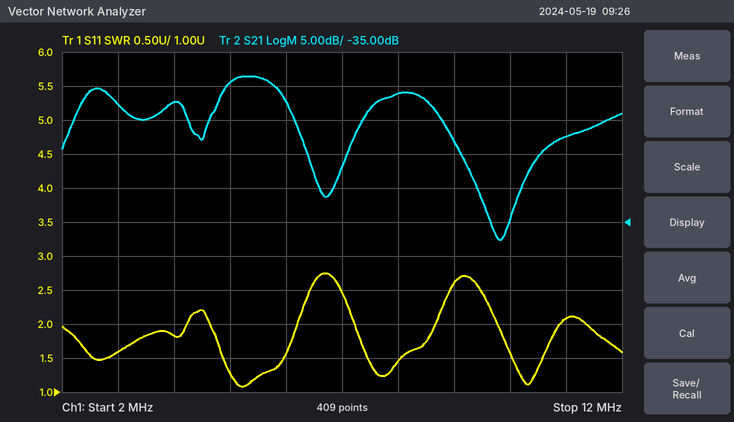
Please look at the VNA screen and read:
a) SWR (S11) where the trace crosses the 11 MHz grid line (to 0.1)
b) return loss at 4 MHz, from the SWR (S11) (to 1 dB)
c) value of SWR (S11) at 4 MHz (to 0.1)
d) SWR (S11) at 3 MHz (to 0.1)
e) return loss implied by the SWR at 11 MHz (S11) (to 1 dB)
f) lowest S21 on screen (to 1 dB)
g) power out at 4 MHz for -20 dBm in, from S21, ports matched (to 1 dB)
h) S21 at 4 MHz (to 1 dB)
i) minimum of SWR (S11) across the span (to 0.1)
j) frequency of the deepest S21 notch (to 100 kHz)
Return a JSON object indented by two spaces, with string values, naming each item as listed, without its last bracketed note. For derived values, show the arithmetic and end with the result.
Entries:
{
  "SWR (S11) where the trace crosses the 11 MHz grid line": "2.1",
  "return loss at 4 MHz, from the SWR (S11)": "−20 log10((1.8 − 1)/(1.8 + 1)) ≈ 11 dB",
  "value of SWR (S11) at 4 MHz": "1.8",
  "SWR (S11) at 3 MHz": "1.6",
  "return loss implied by the SWR at 11 MHz (S11)": "−20 log10((2.1 − 1)/(2.1 + 1)) ≈ 9 dB",
  "lowest S21 on screen": "-38 dB",
  "power out at 4 MHz for -20 dBm in, from S21, ports matched": "-20 dBm + (-17 dB) = -37 dBm",
  "S21 at 4 MHz": "-17 dB",
  "minimum of SWR (S11) across the span": "1.1",
  "frequency of the deepest S21 notch": "9.8 MHz"
}
